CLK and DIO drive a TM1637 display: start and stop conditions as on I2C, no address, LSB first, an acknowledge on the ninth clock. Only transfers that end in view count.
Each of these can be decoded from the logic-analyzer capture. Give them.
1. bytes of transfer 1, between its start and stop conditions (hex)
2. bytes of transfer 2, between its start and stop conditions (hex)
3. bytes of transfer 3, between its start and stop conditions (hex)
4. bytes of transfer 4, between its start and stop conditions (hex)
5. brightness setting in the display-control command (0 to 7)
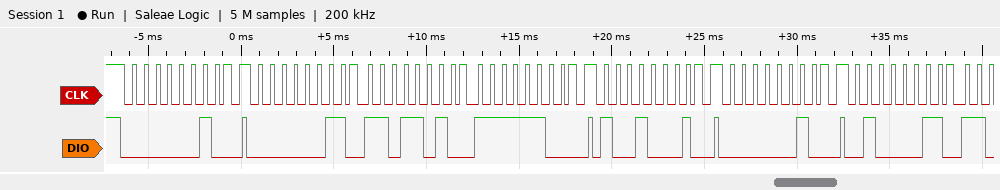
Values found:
40
C0 5B 3F
89
40
1
